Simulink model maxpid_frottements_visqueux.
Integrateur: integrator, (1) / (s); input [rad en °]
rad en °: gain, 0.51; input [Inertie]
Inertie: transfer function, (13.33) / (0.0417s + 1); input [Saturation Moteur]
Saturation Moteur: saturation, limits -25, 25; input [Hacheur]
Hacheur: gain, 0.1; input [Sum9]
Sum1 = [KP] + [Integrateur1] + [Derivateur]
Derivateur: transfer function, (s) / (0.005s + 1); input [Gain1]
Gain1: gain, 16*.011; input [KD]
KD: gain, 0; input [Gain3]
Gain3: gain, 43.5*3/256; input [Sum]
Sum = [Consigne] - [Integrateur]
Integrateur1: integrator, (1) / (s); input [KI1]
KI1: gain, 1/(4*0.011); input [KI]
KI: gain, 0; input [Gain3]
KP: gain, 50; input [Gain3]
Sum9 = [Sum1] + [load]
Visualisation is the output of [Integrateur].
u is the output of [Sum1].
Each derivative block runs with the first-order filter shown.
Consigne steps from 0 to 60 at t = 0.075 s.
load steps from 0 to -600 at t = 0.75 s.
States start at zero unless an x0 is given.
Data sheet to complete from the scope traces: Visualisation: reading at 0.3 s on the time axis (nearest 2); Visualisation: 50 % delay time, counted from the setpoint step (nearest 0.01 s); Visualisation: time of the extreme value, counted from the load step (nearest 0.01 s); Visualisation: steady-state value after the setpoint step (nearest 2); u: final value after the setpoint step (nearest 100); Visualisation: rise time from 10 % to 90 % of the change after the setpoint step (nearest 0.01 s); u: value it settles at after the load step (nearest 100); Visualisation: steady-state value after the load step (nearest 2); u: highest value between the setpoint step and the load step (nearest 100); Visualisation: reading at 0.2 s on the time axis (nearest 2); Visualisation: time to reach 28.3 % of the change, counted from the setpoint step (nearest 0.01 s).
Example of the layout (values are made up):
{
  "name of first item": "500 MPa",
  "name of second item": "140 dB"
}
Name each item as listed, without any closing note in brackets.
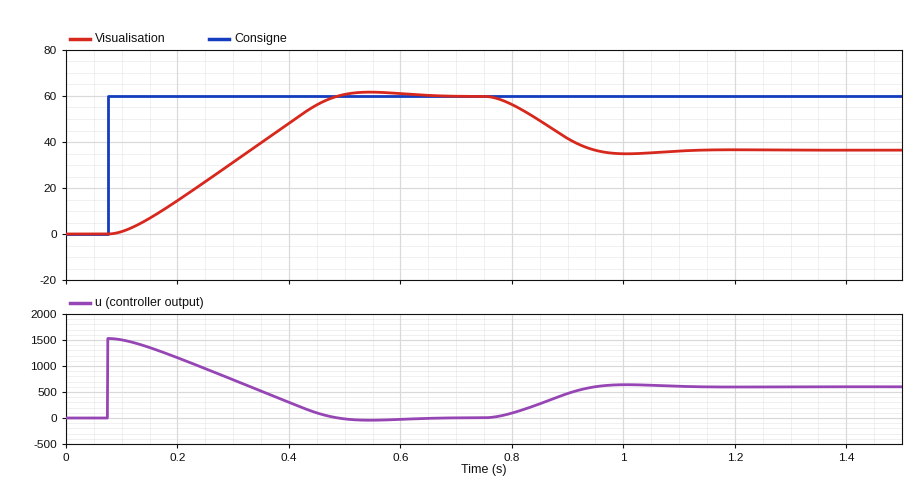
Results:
{
  "Visualisation: reading at 0.3 s on the time axis": "32",
  "Visualisation: 50 % delay time, counted from the setpoint step": "0.22 s",
  "Visualisation: time of the extreme value, counted from the load step": "0.26 s",
  "Visualisation: steady-state value after the setpoint step": "60",
  "u: final value after the setpoint step": "0",
  "Visualisation: rise time from 10 % to 90 % of the change after the setpoint step": "0.29 s",
  "u: value it settles at after the load step": "600",
  "Visualisation: steady-state value after the load step": "36",
  "u: highest value between the setpoint step and the load step": "1500",
  "Visualisation: reading at 0.2 s on the time axis": "14",
  "Visualisation: time to reach 28.3 % of the change, counted from the setpoint step": "0.14 s"
}
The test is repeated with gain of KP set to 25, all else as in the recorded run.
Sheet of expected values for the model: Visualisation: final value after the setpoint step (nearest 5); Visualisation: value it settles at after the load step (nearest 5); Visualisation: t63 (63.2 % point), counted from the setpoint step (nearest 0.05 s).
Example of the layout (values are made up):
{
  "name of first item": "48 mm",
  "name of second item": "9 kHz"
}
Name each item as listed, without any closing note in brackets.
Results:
{
  "Visualisation: final value after the setpoint step": "60",
  "Visualisation: value it settles at after the load step": "15",
  "Visualisation: t63 (63.2 % point), counted from the setpoint step": "0.25 s"
}
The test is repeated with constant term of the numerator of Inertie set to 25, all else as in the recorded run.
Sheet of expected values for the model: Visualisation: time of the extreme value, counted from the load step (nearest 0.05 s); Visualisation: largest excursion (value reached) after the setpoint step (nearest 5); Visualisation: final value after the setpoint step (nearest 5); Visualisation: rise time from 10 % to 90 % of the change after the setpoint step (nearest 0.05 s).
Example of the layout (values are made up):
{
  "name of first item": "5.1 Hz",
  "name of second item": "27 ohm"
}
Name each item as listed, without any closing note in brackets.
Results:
{
  "Visualisation: time of the extreme value, counted from the load step": "0.15 s",
  "Visualisation: largest excursion (value reached) after the setpoint step": "65",
  "Visualisation: final value after the setpoint step": "60",
  "Visualisation: rise time from 10 % to 90 % of the change after the setpoint step": "0.15 s"
}
